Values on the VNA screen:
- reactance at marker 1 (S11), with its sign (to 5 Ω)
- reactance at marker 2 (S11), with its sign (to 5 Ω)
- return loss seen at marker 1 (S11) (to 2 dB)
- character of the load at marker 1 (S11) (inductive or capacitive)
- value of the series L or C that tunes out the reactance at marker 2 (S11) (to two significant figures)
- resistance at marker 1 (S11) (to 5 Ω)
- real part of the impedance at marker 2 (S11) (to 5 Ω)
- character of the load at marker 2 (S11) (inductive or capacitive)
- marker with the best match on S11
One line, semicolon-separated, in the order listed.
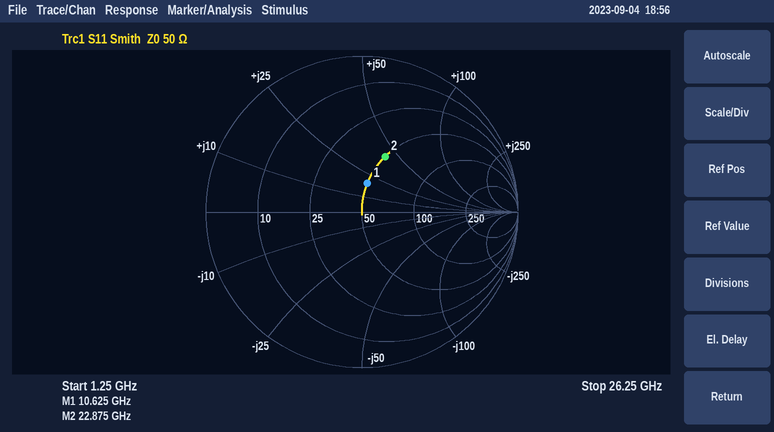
+20 Ω; +40 Ω; 14 dB; inductive; 170 fF; 50 Ω; 50 Ω; inductive; marker 1
